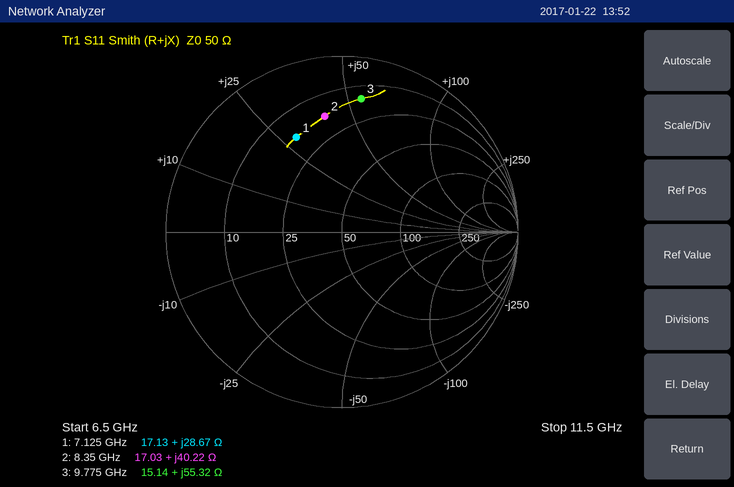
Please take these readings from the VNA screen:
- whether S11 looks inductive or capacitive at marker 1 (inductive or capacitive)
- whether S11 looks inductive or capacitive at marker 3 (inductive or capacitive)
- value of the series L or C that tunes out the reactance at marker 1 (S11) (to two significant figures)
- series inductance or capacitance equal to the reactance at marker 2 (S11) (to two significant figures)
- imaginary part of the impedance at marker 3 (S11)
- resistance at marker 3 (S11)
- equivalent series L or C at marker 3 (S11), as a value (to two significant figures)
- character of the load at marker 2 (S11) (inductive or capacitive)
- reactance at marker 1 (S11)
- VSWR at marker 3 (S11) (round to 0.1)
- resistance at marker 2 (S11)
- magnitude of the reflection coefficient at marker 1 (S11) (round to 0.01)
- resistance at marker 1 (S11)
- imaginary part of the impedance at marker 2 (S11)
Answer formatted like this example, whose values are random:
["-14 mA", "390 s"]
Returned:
["inductive", "inductive", "780 fF", "770 pH", "+55.32 Ω", "15.14 Ω", "900 pH", "inductive", "+28.67 Ω", "7.5", "17.03 Ω", "0.60", "17.13 Ω", "+40.22 Ω"]
